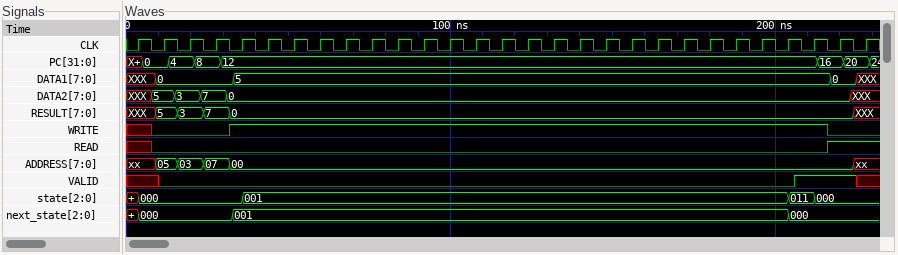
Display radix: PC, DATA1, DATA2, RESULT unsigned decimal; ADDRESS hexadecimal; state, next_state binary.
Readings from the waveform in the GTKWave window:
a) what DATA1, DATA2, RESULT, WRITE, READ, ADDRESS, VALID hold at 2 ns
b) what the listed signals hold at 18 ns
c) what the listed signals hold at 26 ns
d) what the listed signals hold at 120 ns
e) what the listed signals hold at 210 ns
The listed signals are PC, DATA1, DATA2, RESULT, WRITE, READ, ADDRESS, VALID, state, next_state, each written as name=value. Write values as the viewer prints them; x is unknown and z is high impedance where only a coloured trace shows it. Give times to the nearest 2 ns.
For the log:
DATA1=XXX, DATA2=XXX, RESULT=XXX, WRITE=x, READ=x, ADDRESS=xx, VALID=x
PC=4, DATA1=0, DATA2=3, RESULT=3, WRITE=0, READ=0, ADDRESS=03, VALID=0, state=000, next_state=000
PC=8, DATA1=0, DATA2=7, RESULT=7, WRITE=0, READ=0, ADDRESS=07, VALID=0, state=000, next_state=000
PC=12, DATA1=5, DATA2=0, RESULT=0, WRITE=1, READ=0, ADDRESS=00, VALID=0, state=001, next_state=001
PC=12, DATA1=5, DATA2=0, RESULT=0, WRITE=1, READ=0, ADDRESS=00, VALID=1, state=011, next_state=000
